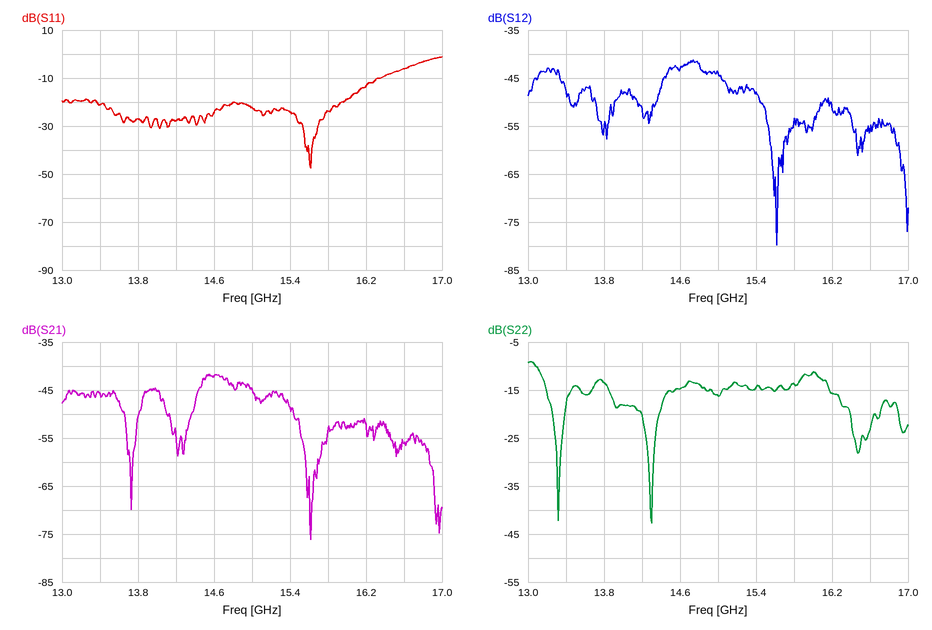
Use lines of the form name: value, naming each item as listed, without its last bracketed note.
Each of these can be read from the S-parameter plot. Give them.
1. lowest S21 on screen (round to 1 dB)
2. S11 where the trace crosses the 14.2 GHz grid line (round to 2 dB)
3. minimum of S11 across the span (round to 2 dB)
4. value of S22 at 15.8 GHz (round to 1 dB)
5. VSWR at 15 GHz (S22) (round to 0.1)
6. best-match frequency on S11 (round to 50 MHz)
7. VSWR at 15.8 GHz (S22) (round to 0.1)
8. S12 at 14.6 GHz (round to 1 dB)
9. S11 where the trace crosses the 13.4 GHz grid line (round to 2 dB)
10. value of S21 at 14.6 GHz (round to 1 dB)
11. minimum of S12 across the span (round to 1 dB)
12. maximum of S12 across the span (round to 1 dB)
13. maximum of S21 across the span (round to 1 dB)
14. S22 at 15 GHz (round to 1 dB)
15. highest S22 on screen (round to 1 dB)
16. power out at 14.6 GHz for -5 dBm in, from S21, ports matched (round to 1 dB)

lowest S21 on screen: -76 dB
S11 where the trace crosses the 14.2 GHz grid line: -28 dB
minimum of S11 across the span: -48 dB
value of S22 at 15.8 GHz: -14 dB
VSWR at 15 GHz (S22): 1.4
best-match frequency on S11: 15.60 GHz
VSWR at 15.8 GHz (S22): 1.5
S12 at 14.6 GHz: -43 dB
S11 where the trace crosses the 13.4 GHz grid line: -22 dB
value of S21 at 14.6 GHz: -42 dB
minimum of S12 across the span: -80 dB
maximum of S12 across the span: -41 dB
maximum of S21 across the span: -42 dB
S22 at 15 GHz: -16 dB
highest S22 on screen: -9 dB
power out at 14.6 GHz for -5 dBm in, from S21, ports matched: -47 dBm
